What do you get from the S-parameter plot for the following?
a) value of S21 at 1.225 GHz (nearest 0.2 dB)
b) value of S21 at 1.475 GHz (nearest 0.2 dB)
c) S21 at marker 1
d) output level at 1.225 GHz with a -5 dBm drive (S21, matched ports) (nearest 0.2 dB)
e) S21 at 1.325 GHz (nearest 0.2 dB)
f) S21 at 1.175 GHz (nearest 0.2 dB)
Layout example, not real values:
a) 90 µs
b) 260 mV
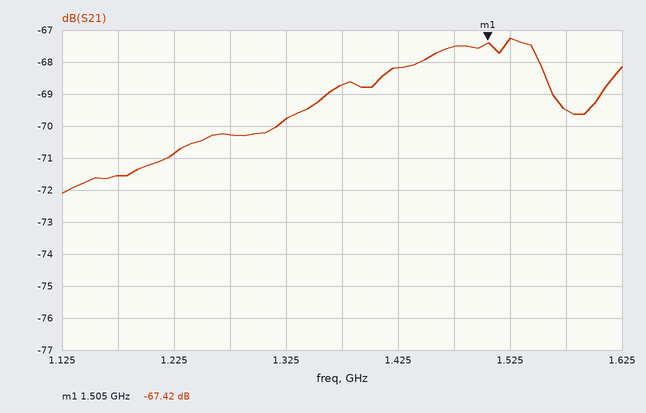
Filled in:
a) -70.8 dB
b) -67.6 dB
c) -67.42 dB
d) -75.8 dBm
e) -69.8 dB
f) -71.6 dB
